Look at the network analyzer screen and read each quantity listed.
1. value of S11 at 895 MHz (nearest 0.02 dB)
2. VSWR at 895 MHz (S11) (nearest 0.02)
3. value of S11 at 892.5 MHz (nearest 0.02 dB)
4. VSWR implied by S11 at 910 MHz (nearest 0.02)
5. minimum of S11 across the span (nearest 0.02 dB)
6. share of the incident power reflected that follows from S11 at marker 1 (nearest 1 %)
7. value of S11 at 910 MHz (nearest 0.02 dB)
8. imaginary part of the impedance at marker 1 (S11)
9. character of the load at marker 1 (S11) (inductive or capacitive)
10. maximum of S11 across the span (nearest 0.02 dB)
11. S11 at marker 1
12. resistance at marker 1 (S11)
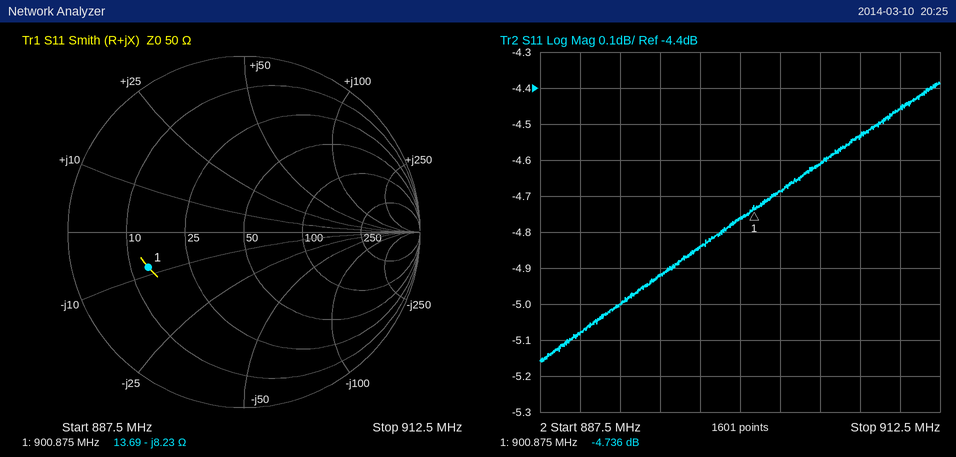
-4.92 dB
3.62
-5.00 dB
3.98
-5.16 dB
34 %
-4.46 dB
-8.23 Ω
capacitive
-4.38 dB
-4.736 dB
13.69 Ω
